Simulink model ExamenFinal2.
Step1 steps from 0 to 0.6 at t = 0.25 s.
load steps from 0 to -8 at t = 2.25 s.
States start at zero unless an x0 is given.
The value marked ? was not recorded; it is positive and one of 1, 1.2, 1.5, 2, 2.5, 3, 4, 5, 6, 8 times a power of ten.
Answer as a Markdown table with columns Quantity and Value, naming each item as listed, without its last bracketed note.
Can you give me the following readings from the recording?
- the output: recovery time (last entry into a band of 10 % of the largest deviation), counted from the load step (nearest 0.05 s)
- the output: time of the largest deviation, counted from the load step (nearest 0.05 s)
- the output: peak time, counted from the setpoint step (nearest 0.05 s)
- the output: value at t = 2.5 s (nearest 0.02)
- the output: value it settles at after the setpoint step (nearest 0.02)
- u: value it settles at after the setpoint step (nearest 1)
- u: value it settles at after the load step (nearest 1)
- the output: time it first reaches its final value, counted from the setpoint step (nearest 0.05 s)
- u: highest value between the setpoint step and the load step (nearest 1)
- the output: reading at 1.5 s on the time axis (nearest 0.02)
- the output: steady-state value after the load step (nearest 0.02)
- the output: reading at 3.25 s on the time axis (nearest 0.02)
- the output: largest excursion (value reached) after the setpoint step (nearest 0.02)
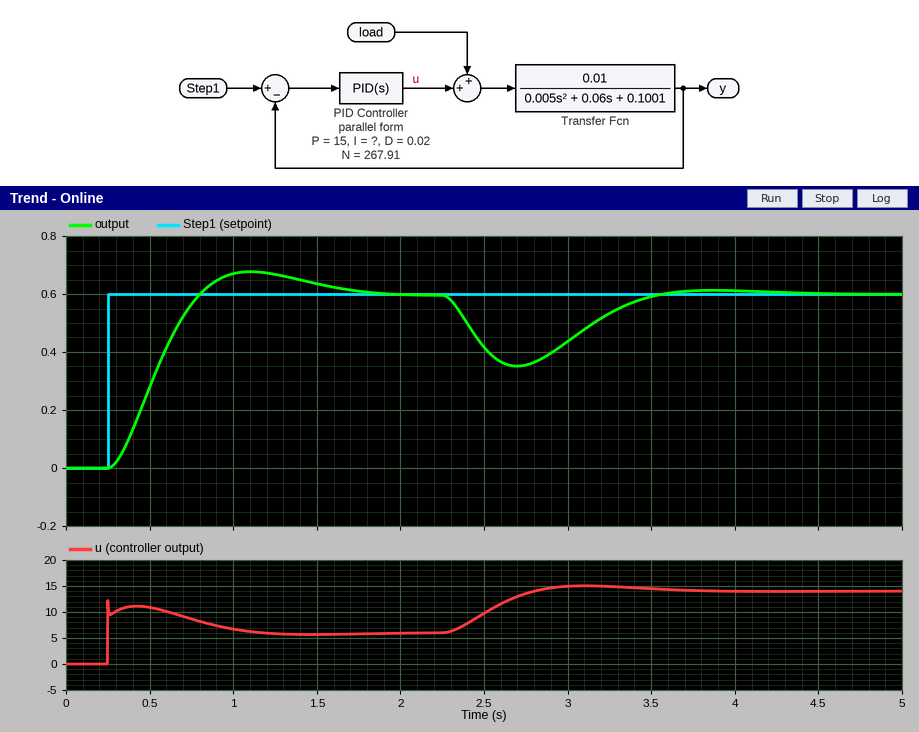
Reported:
| Quantity | Value |
|---|---|
| the output: recovery time (last entry into a band of 10 % of the largest deviation), counted from the load step | 1.15 s |
| the output: time of the largest deviation, counted from the load step | 0.45 s |
| the output: peak time, counted from the setpoint step | 0.85 s |
| the output: value at t = 2.5 s | 0.42 |
| the output: value it settles at after the setpoint step | 0.60 |
| u: value it settles at after the setpoint step | 6 |
| u: value it settles at after the load step | 14 |
| the output: time it first reaches its final value, counted from the setpoint step | 0.55 s |
| u: highest value between the setpoint step and the load step | 12 |
| the output: reading at 1.5 s on the time axis | 0.64 |
| the output: steady-state value after the load step | 0.60 |
| the output: reading at 3.25 s on the time axis | 0.54 |
| the output: largest excursion (value reached) after the setpoint step | 0.68 |
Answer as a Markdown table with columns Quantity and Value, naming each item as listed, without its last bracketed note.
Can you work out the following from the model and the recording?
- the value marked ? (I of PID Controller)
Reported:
| Quantity | Value |
|---|---|
| the value marked ? | 50 |
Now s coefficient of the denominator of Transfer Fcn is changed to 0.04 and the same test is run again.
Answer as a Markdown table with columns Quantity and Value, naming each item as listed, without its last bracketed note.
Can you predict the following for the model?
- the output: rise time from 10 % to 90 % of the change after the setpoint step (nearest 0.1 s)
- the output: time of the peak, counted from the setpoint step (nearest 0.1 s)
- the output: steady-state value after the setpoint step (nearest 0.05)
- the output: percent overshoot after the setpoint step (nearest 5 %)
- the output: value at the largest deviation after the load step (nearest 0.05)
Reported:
| Quantity | Value |
|---|---|
| the output: rise time from 10 % to 90 % of the change after the setpoint step | 0.3 s |
| the output: time of the peak, counted from the setpoint step | 0.6 s |
| the output: steady-state value after the setpoint step | 0.60 |
| the output: percent overshoot after the setpoint step | 15 % |
| the output: value at the largest deviation after the load step | 0.30 |
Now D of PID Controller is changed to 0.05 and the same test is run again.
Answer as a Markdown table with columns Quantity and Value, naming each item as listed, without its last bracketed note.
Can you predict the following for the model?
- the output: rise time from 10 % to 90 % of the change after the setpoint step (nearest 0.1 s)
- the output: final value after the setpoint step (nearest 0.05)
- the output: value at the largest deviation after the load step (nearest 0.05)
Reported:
| Quantity | Value |
|---|---|
| the output: rise time from 10 % to 90 % of the change after the setpoint step | 0.4 s |
| the output: final value after the setpoint step | 0.60 |
| the output: value at the largest deviation after the load step | 0.35 |
